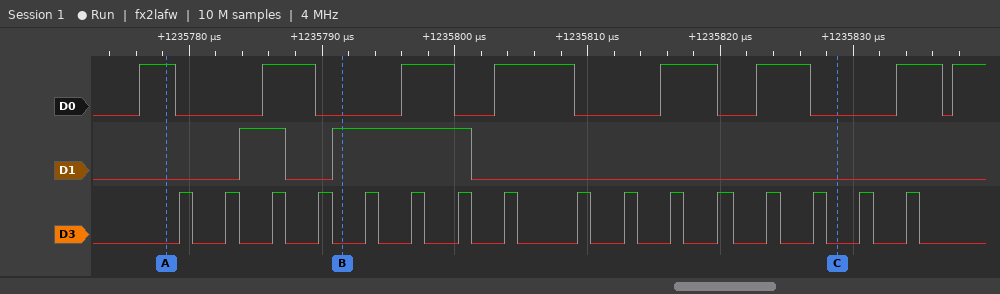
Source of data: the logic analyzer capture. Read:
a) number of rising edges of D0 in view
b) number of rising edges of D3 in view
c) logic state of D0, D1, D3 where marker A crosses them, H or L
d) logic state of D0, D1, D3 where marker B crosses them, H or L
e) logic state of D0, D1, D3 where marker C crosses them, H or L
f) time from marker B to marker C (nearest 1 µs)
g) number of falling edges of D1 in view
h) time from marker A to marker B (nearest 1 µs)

8
16
D0=H, D1=L, D3=L
D0=L, D1=H, D3=L
D0=L, D1=L, D3=L
37 µs
2
13 µs
